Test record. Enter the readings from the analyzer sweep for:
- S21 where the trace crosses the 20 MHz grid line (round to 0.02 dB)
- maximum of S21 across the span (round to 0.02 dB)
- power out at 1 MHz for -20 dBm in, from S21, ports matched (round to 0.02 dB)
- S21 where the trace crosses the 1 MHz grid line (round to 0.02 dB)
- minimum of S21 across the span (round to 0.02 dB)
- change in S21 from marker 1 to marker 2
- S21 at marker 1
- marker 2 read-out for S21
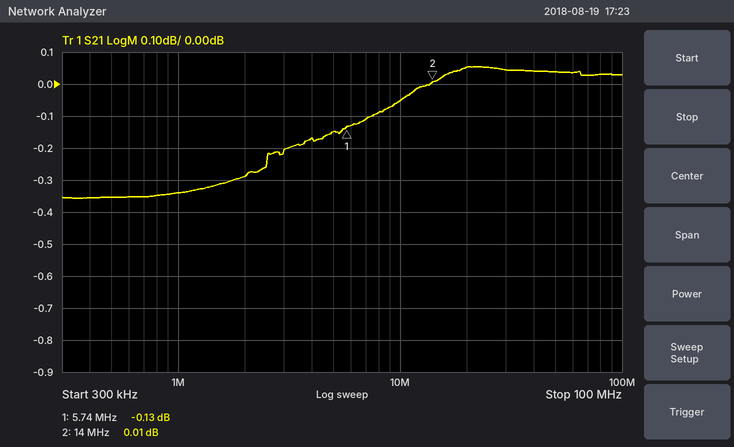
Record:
0.06 dB
0.06 dB
-20.34 dBm
-0.34 dB
-0.36 dB
0.14 dB
-0.13 dB
0.01 dB
